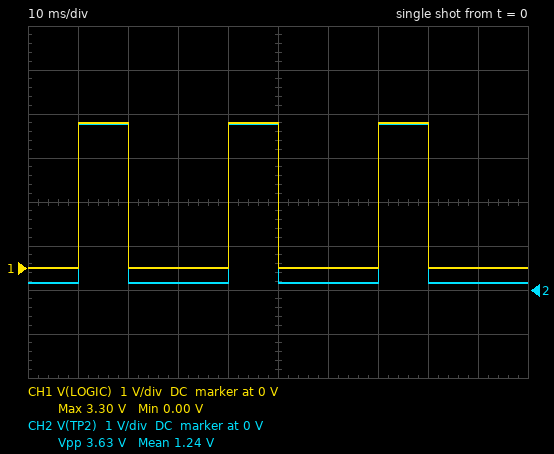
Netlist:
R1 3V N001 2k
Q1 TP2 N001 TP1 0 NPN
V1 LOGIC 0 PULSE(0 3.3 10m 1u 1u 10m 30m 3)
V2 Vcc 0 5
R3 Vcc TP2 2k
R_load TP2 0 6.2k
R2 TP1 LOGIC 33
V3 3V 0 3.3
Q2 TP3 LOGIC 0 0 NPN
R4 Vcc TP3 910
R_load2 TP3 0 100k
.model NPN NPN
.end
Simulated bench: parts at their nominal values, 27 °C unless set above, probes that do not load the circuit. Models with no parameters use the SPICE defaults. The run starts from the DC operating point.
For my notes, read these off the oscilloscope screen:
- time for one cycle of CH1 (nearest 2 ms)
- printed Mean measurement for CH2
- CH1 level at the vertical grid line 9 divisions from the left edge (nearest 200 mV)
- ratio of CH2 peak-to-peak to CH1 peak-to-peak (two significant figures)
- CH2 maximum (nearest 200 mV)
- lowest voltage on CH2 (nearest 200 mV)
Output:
30 ms
1.24 V
0 V
1.1
3.8 V
200 mV
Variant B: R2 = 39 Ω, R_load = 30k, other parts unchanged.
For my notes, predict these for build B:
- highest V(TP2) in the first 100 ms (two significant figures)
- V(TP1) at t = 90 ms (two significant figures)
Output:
4.7 V
140 mV
